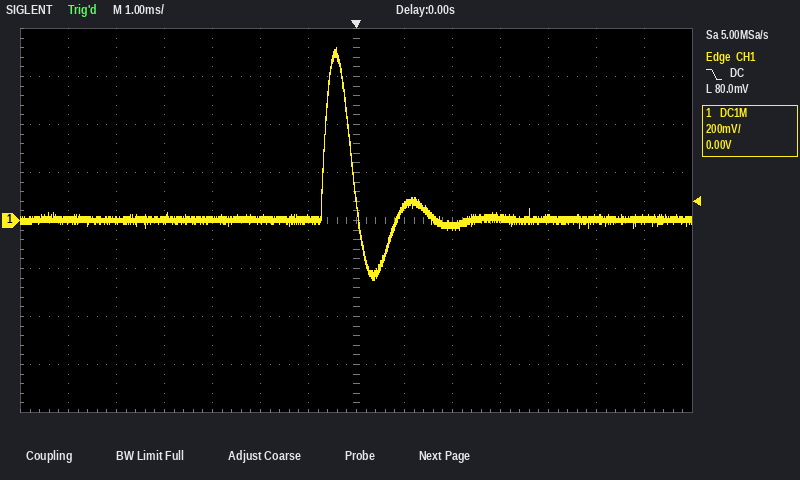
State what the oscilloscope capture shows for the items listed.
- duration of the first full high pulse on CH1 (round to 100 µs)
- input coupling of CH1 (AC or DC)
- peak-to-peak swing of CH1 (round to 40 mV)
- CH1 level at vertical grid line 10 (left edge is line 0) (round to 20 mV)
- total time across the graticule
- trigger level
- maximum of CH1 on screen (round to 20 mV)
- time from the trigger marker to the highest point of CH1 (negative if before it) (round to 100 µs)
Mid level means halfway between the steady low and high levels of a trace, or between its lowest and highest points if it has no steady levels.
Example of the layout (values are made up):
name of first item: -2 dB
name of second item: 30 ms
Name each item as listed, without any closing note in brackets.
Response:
duration of the first full high pulse on CH1: 600 µs
input coupling of CH1: DC
peak-to-peak swing of CH1: 960 mV
CH1 level at vertical grid line 10 (left edge is line 0): 0 mV
total time across the graticule: 14 ms
trigger level: 80.0 mV
maximum of CH1 on screen: 720 mV
time from the trigger marker to the highest point of CH1 (negative if before it): -400 µs
